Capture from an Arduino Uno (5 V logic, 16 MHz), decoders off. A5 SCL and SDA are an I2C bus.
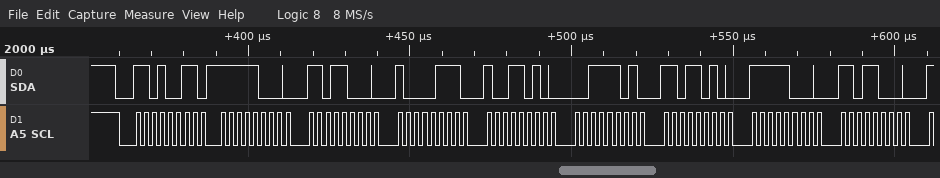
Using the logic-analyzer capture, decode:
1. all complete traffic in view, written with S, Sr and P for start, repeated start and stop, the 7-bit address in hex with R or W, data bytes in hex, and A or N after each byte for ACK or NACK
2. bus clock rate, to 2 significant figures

S 69R A F8 A D8 A 87 A 9A A 3D A DA A F8 A D8 A
400 kHz
